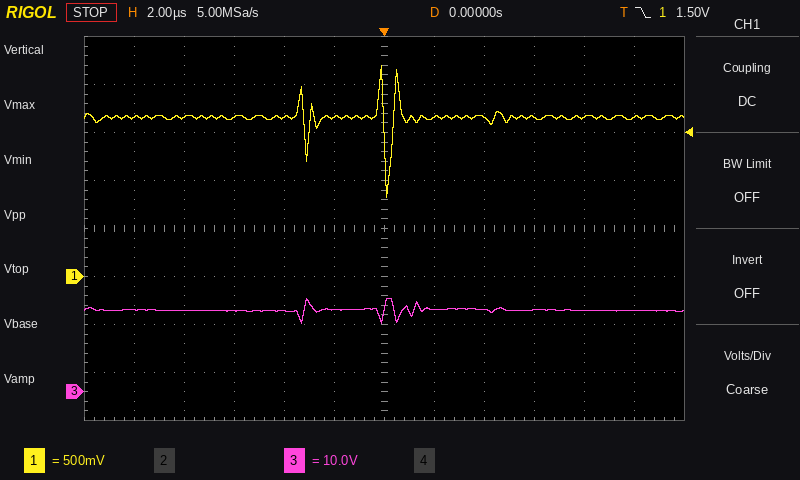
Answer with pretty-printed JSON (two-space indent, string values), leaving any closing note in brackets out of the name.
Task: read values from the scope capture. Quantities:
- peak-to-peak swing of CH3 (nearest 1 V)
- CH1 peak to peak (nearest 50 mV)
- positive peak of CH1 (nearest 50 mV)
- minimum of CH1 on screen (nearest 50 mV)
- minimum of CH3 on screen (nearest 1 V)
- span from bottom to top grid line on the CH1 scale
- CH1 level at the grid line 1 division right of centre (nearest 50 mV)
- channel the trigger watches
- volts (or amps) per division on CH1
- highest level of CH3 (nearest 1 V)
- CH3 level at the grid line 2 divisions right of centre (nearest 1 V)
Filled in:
{
  "peak-to-peak swing of CH3": "5 V",
  "CH1 peak to peak": "1.40 V",
  "positive peak of CH1": "2.20 V",
  "minimum of CH1 on screen": "800 mV",
  "minimum of CH3 on screen": "14 V",
  "span from bottom to top grid line on the CH1 scale": "4 V",
  "CH1 level at the grid line 1 division right of centre": "1.65 V",
  "channel the trigger watches": "CH1",
  "volts (or amps) per division on CH1": "500 mV",
  "highest level of CH3": "19 V",
  "CH3 level at the grid line 2 divisions right of centre": "17 V"
}
